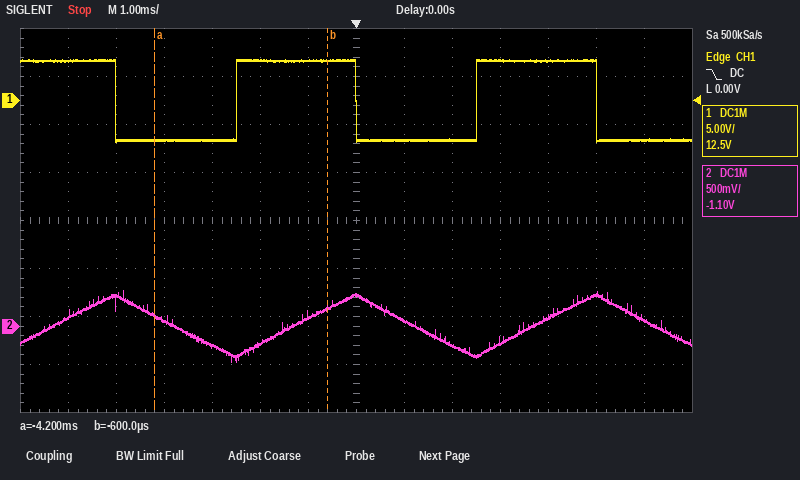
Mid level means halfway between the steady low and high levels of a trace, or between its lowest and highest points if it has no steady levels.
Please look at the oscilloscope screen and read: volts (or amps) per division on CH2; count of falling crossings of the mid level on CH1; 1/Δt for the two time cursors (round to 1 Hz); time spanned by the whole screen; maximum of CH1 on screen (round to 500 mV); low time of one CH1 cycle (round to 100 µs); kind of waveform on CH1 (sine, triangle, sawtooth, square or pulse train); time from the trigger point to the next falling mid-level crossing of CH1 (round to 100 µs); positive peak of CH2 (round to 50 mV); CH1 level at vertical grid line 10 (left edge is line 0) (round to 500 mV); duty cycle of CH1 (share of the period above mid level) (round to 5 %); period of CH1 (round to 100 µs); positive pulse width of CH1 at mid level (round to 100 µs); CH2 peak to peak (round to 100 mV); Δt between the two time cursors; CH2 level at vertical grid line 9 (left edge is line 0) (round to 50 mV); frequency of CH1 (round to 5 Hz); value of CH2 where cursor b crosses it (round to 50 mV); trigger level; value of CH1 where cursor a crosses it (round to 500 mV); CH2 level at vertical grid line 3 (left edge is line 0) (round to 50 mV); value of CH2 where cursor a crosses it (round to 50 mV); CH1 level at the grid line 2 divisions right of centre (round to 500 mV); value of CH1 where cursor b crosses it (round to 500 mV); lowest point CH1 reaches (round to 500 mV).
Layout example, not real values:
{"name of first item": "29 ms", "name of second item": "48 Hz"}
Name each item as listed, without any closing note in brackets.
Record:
{"volts (or amps) per division on CH2": "500 mV", "count of falling crossings of the mid level on CH1": "3", "1/Δt for the two time cursors": "278 Hz", "time spanned by the whole screen": "14 ms", "maximum of CH1 on screen": "4.5 V", "low time of one CH1 cycle": "2.5 ms", "kind of waveform on CH1": "square", "time from the trigger point to the next falling mid-level crossing of CH1": "5.0 ms", "positive peak of CH2": "350 mV", "CH1 level at vertical grid line 10 (left edge is line 0)": "4.0 V", "duty cycle of CH1 (share of the period above mid level)": "50 %", "period of CH1": "5.0 ms", "positive pulse width of CH1 at mid level": "2.5 ms", "CH2 peak to peak": "700 mV", "Δt between the two time cursors": "3.6 ms", "CH2 level at vertical grid line 9 (left edge is line 0)": "-200 mV", "frequency of CH1": "200 Hz", "value of CH2 where cursor b crosses it": "200 mV", "trigger level": "0.00 V", "value of CH1 where cursor a crosses it": "-4.0 V", "CH2 level at vertical grid line 3 (left edge is line 0)": "50 mV", "value of CH2 where cursor a crosses it": "100 mV", "CH1 level at the grid line 2 divisions right of centre": "-4.0 V", "value of CH1 where cursor b crosses it": "4.0 V", "lowest point CH1 reaches": "-4.5 V"}
